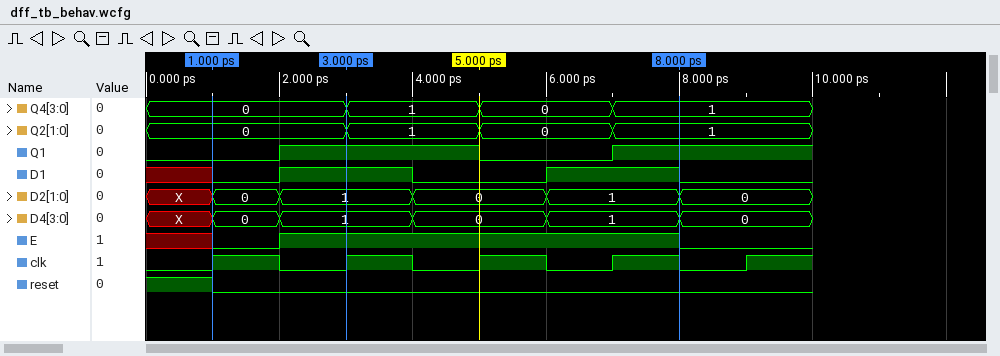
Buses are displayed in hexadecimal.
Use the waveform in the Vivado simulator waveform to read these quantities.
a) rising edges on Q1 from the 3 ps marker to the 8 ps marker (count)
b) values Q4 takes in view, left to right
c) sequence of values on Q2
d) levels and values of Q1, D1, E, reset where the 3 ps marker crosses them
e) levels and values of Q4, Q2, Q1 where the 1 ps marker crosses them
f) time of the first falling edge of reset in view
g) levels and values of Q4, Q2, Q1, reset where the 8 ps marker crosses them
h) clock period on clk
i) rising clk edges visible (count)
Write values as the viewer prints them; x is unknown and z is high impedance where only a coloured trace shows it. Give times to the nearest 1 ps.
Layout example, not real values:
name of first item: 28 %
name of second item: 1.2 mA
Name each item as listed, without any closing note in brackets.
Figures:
rising edges on Q1 from the 3 ps marker to the 8 ps marker: 1
values Q4 takes in view, left to right: 0, 1, 0, 1
sequence of values on Q2: 0, 1, 0, 1
levels and values of Q1, D1, E, reset where the 3 ps marker crosses them: Q1=1, D1=1, E=1, reset=0
levels and values of Q4, Q2, Q1 where the 1 ps marker crosses them: Q4=0, Q2=0, Q1=0
time of the first falling edge of reset in view: 1 ps
levels and values of Q4, Q2, Q1, reset where the 8 ps marker crosses them: Q4=1, Q2=1, Q1=1, reset=0
clock period on clk: 2 ps
rising clk edges visible: 5
